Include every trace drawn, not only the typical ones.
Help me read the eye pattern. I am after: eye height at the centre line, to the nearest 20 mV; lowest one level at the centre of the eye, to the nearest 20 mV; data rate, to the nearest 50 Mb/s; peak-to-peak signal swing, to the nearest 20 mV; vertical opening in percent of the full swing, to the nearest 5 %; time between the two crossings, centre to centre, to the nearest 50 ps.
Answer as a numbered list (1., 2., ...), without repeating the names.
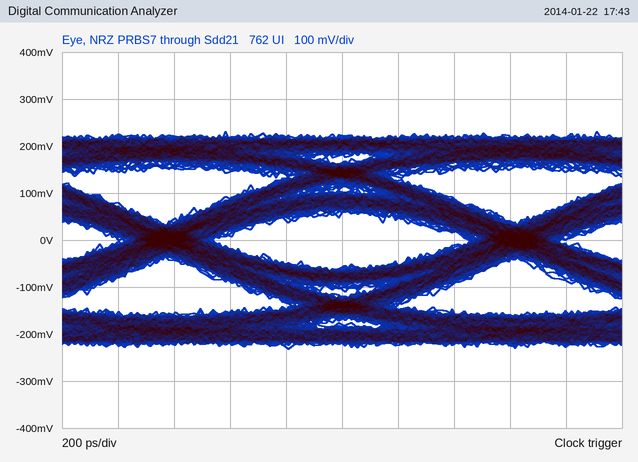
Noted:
1. 120 mV
2. 60 mV
3. 800 Mb/s
4. 460 mV
5. 25 %
6. 1.25 ns
